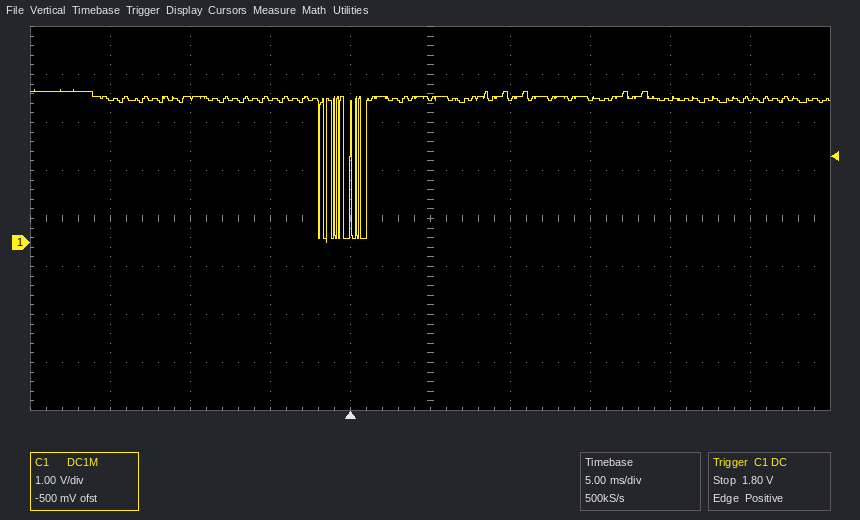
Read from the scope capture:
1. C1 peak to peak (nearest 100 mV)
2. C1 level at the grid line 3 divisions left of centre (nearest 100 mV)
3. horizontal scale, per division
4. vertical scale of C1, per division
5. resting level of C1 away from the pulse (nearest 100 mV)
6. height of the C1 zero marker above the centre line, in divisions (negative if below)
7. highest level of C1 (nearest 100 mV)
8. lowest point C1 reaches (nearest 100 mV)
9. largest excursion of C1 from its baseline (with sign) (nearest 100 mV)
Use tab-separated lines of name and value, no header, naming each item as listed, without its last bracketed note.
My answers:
C1 peak to peak	3.2 V
C1 level at the grid line 3 divisions left of centre	3.0 V
horizontal scale, per division	5 ms
vertical scale of C1, per division	1 V
resting level of C1 away from the pulse	3.0 V
height of the C1 zero marker above the centre line, in divisions	-0.5 div
highest level of C1	3.2 V
lowest point C1 reaches	0.0 V
largest excursion of C1 from its baseline (with sign)	-3.0 V
